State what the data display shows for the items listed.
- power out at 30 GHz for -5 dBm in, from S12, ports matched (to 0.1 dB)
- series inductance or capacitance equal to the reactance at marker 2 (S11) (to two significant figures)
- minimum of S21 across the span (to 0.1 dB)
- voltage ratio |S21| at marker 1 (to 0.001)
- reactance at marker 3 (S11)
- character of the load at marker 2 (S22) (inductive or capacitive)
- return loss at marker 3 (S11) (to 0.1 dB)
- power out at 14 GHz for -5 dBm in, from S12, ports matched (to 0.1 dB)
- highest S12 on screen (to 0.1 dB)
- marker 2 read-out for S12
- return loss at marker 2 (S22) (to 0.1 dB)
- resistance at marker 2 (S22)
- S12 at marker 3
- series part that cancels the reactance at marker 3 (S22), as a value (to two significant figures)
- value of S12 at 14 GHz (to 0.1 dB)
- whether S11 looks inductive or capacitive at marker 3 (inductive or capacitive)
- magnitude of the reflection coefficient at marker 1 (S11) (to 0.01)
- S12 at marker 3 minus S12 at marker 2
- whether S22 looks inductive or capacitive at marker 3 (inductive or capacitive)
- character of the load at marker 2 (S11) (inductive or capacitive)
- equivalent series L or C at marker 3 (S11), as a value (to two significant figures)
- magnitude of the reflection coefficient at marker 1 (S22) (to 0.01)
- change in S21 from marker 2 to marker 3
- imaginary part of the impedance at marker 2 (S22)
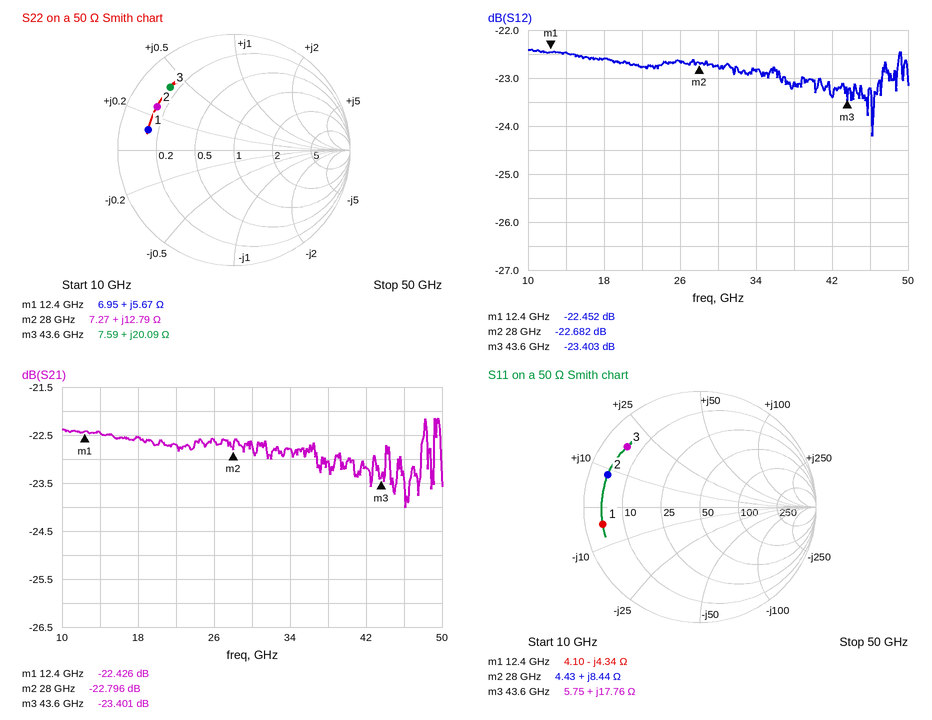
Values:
-27.8 dBm
48 pH
-24.0 dB
0.076
+17.76 Ω
inductive
1.8 dB
-27.5 dBm
-22.4 dB
-22.682 dB
2.4 dB
7.27 Ω
-23.403 dB
180 fF
-22.5 dB
inductive
0.85
-0.721 dB
inductive
inductive
65 pH
0.76
-0.605 dB
+12.79 Ω
